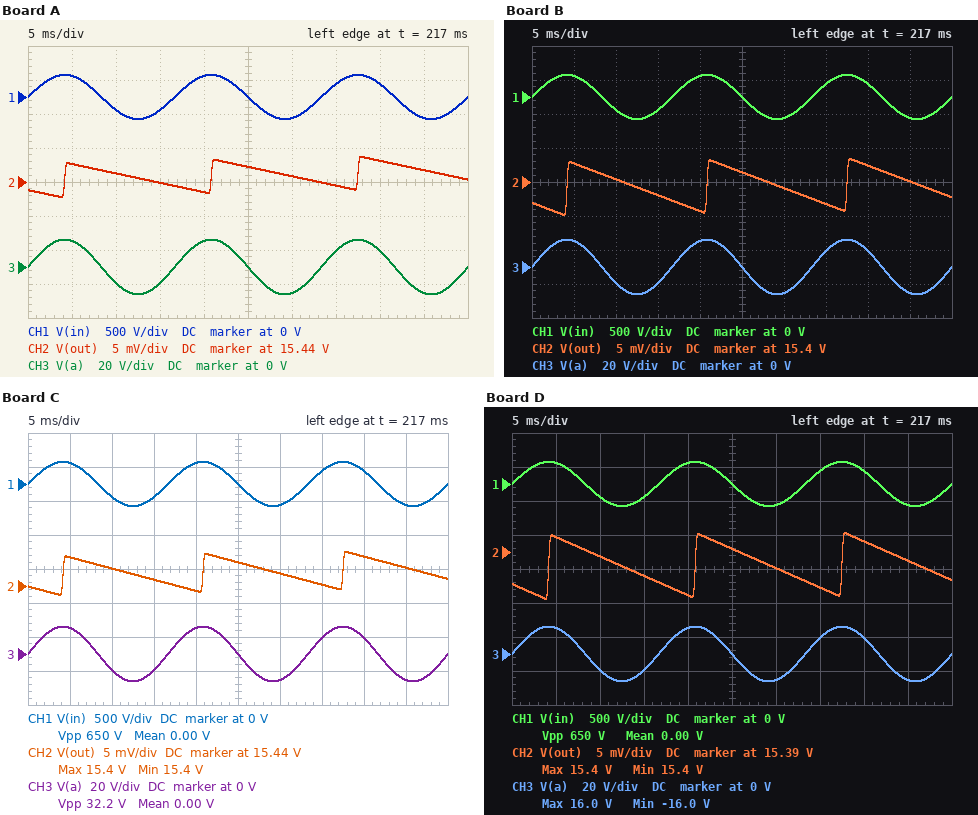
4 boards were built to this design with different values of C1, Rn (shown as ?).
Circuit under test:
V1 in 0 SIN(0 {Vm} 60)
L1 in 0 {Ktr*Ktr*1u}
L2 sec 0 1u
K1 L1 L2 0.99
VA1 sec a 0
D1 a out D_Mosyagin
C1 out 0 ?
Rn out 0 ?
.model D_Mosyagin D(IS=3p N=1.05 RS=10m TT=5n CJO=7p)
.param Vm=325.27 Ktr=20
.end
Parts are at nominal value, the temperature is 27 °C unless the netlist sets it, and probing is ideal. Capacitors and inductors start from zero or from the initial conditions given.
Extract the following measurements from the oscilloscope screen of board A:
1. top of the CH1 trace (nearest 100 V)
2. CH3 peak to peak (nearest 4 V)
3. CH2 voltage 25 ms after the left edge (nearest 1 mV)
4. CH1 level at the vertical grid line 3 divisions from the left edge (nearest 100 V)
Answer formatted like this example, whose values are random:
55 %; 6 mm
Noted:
300 V; 32 V; 15.442 V; -200 V
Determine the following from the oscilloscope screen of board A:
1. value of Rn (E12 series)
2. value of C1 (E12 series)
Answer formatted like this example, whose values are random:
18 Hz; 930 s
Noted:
10 kΩ; 5.6 mF
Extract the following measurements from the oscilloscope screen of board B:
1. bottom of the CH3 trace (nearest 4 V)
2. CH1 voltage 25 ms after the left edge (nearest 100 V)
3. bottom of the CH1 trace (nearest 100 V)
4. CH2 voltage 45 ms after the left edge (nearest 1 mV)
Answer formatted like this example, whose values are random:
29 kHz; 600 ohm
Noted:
-16 V; 0 V; -300 V; 15.400 V
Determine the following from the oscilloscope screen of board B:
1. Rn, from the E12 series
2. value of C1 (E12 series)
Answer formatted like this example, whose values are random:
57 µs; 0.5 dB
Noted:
2.2 kΩ; 15 mF
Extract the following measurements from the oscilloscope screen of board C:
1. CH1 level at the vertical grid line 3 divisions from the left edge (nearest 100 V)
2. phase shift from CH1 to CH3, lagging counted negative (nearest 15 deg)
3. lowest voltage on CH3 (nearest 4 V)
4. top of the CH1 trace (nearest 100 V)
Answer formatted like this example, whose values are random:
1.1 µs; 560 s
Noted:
-200 V; 0 deg; -16 V; 300 V
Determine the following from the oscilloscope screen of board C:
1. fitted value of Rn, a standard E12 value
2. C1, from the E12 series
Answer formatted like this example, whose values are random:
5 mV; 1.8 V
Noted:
10 kΩ; 4.7 mF
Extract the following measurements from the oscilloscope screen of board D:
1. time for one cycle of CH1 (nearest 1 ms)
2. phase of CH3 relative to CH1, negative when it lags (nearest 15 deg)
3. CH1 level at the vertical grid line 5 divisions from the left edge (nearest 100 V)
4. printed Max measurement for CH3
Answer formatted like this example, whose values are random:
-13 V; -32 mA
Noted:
17 ms; 0 deg; 0 V; 16.0 V
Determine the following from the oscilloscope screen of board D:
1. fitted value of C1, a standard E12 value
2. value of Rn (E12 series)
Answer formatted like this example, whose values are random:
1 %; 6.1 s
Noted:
18 mF; 1.5 kΩ
